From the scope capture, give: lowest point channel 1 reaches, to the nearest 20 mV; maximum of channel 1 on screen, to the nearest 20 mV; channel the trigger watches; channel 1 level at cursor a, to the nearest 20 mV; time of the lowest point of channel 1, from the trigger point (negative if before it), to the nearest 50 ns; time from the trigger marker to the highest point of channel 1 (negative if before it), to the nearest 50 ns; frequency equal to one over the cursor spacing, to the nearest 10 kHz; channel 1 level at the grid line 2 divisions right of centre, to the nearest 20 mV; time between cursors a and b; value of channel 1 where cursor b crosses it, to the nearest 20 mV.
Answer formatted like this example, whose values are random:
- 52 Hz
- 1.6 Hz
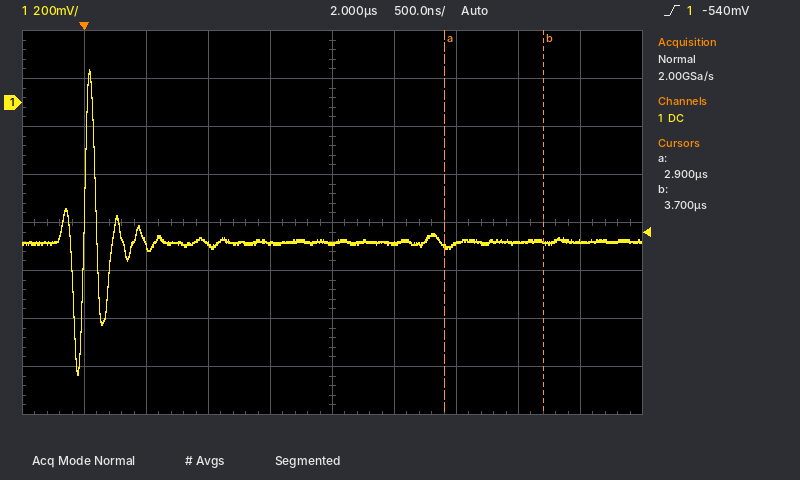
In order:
- -1.14 V
- 140 mV
- channel 1
- -600 mV
- -50 ns
- +50 ns
- 1.25 MHz
- -580 mV
- 800 ns
- -580 mV
